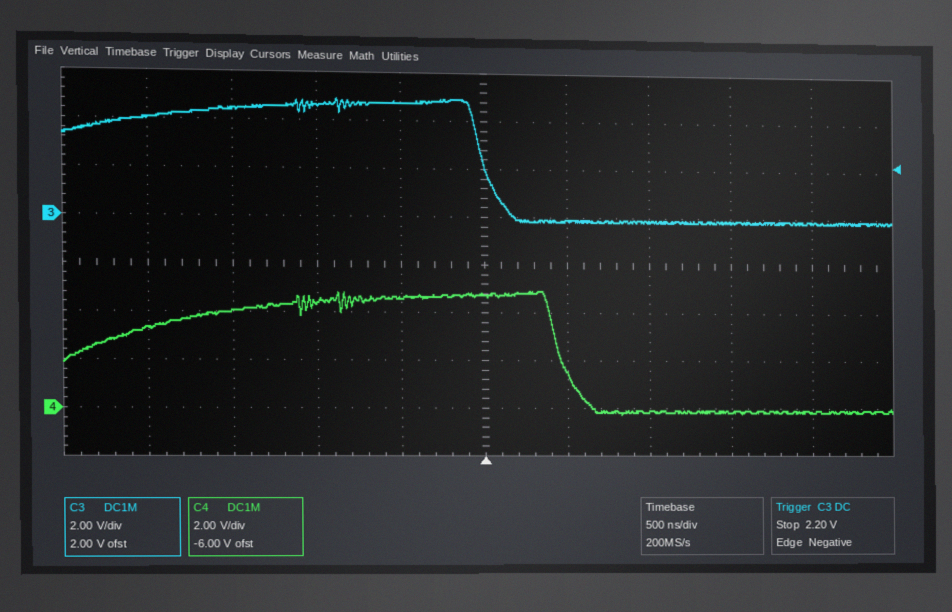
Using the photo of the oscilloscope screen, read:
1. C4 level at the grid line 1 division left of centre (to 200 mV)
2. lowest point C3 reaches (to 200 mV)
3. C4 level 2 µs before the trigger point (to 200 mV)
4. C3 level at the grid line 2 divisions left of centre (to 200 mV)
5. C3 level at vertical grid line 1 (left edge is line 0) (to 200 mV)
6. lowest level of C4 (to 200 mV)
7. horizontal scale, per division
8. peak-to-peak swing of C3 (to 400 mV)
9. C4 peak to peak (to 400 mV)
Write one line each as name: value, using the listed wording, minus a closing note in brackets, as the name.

C4 level at the grid line 1 division left of centre: 4.6 V
lowest point C3 reaches: -200 mV
C4 level 2 µs before the trigger point: 3.4 V
C3 level at the grid line 2 divisions left of centre: 4.6 V
C3 level at vertical grid line 1 (left edge is line 0): 4.0 V
lowest level of C4: -200 mV
horizontal scale, per division: 500 ns
peak-to-peak swing of C3: 5.2 V
C4 peak to peak: 5.2 V
